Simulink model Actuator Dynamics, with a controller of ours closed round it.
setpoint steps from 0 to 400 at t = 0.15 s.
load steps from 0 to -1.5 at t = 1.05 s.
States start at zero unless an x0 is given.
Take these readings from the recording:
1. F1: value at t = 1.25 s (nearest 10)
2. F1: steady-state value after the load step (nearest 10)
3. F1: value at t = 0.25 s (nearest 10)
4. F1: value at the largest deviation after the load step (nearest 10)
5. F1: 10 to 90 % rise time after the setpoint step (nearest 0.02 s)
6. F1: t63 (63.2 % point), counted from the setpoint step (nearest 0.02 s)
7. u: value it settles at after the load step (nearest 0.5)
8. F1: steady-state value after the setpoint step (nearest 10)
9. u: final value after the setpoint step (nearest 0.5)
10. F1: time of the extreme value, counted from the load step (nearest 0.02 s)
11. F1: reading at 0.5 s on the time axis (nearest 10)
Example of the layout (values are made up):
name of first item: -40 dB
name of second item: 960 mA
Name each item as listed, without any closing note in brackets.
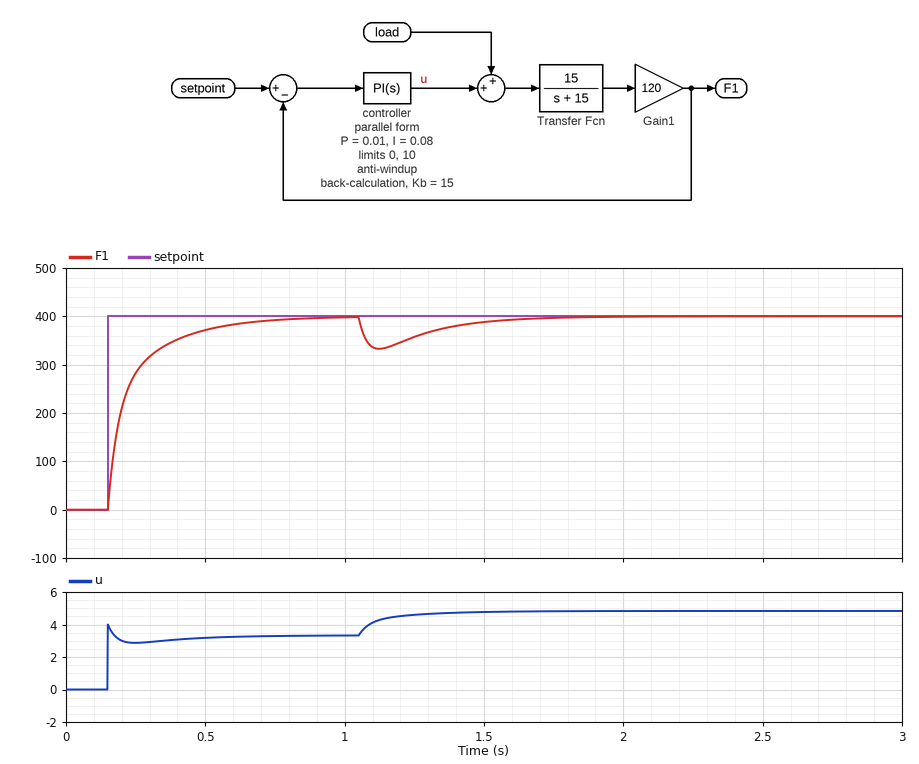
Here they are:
F1: value at t = 1.25 s: 360
F1: steady-state value after the load step: 400
F1: value at t = 0.25 s: 280
F1: value at the largest deviation after the load step: 330
F1: 10 to 90 % rise time after the setpoint step: 0.28 s
F1: t63 (63.2 % point), counted from the setpoint step: 0.08 s
u: value it settles at after the load step: 5.0
F1: steady-state value after the setpoint step: 400
u: final value after the setpoint step: 3.5
F1: time of the extreme value, counted from the load step: 0.08 s
F1: reading at 0.5 s on the time axis: 370
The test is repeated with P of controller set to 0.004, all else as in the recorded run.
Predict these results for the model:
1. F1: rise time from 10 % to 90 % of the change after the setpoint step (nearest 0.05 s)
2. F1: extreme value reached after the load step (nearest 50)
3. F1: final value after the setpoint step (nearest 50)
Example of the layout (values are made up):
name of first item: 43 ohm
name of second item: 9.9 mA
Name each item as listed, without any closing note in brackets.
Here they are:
F1: rise time from 10 % to 90 % of the change after the setpoint step: 0.20 s
F1: extreme value reached after the load step: 300
F1: final value after the setpoint step: 400
